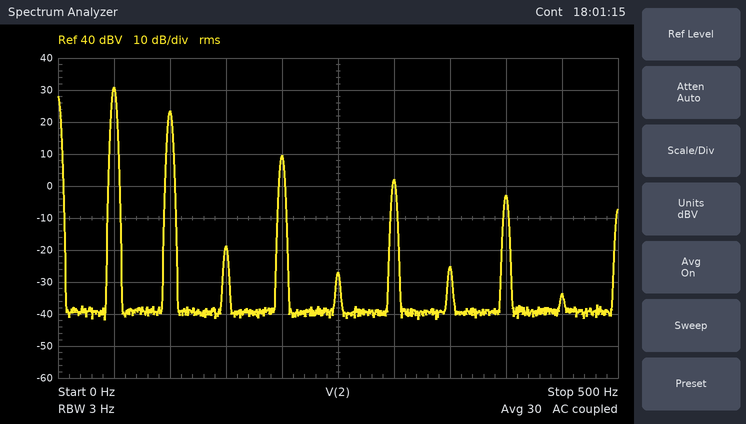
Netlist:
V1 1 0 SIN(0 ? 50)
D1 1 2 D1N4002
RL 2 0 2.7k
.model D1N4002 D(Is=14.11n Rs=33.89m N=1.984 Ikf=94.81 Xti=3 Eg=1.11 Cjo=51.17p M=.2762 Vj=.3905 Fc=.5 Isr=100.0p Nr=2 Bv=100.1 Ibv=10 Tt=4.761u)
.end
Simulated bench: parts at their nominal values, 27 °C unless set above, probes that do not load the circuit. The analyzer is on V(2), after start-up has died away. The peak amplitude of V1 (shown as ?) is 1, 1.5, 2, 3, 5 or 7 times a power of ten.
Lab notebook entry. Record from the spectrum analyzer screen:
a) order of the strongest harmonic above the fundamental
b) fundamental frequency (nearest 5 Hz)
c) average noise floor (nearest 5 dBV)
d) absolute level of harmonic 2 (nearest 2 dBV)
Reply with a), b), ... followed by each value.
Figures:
a) 2
b) 50 Hz
c) -40 dBV
d) 24 dBV
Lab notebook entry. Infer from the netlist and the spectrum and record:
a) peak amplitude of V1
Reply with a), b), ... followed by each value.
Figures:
a) 100 V
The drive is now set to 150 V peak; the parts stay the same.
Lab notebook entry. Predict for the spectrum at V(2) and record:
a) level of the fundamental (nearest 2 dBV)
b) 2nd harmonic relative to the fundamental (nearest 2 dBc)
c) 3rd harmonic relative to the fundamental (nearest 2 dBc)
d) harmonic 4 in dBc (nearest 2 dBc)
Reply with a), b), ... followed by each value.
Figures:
a) 36 dBV
b) -14 dBc
c) -20 dBc
d) -18 dBc
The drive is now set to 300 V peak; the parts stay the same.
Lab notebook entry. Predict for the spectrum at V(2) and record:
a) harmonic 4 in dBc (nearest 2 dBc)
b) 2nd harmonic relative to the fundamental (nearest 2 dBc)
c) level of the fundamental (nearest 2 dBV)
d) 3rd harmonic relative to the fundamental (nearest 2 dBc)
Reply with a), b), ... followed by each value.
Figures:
a) -28 dBc
b) -28 dBc
c) 44 dBV
d) -22 dBc
